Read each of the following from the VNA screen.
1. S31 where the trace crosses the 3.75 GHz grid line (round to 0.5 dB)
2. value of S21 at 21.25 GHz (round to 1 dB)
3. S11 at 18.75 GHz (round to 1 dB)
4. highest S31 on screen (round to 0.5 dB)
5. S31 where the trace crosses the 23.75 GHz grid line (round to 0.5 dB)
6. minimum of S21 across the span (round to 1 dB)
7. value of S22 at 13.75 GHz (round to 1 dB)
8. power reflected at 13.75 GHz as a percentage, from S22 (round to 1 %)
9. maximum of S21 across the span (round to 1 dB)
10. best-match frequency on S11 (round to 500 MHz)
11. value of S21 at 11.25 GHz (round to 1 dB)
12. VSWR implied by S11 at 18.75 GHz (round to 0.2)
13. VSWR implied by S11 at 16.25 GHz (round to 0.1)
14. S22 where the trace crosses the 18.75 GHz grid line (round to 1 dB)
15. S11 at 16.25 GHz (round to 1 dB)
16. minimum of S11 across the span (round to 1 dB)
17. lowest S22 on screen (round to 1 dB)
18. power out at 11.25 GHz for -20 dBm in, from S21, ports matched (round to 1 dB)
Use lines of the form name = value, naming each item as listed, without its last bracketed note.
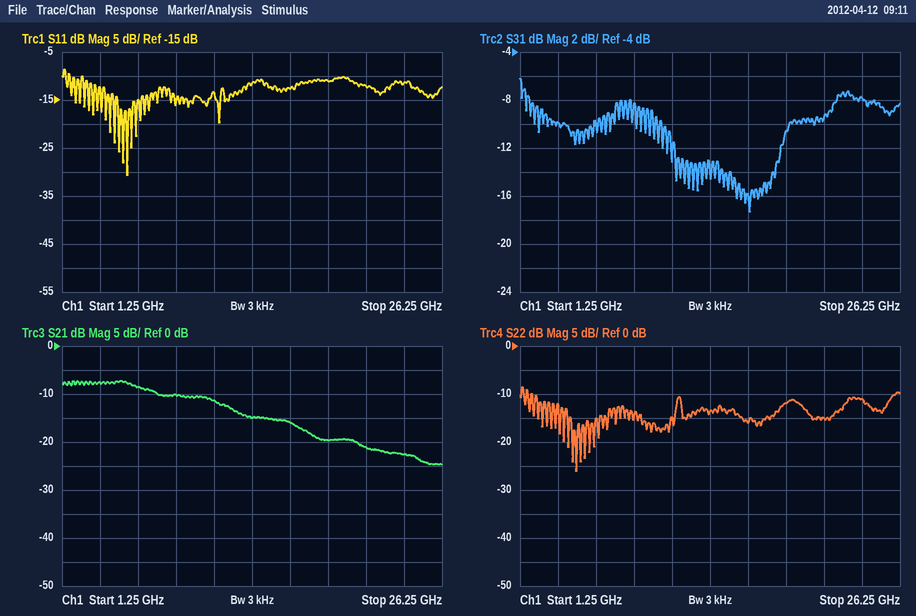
S31 where the trace crosses the 3.75 GHz grid line = -10.0 dB
value of S21 at 21.25 GHz = -21 dB
S11 at 18.75 GHz = -11 dB
highest S31 on screen = -6.0 dB
S31 where the trace crosses the 23.75 GHz grid line = -8.0 dB
minimum of S21 across the span = -25 dB
value of S22 at 13.75 GHz = -14 dB
power reflected at 13.75 GHz as a percentage, from S22 = 4 %
maximum of S21 across the span = -7 dB
best-match frequency on S11 = 5.5 GHz
value of S21 at 11.25 GHz = -11 dB
VSWR implied by S11 at 18.75 GHz = 1.8
VSWR implied by S11 at 16.25 GHz = 1.6
S22 where the trace crosses the 18.75 GHz grid line = -12 dB
S11 at 16.25 GHz = -13 dB
minimum of S11 across the span = -31 dB
lowest S22 on screen = -26 dB
power out at 11.25 GHz for -20 dBm in, from S21, ports matched = -31 dBm
